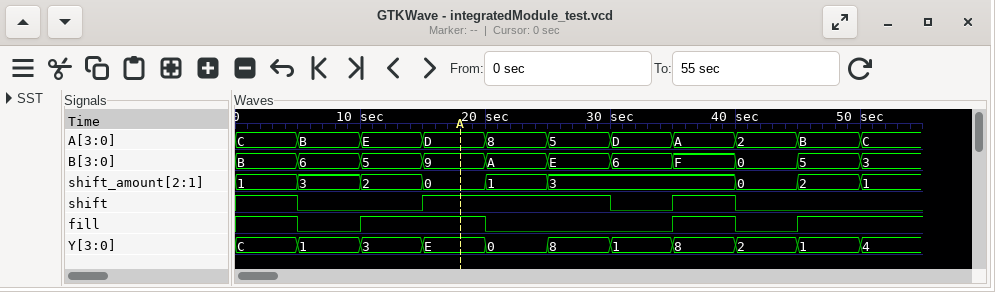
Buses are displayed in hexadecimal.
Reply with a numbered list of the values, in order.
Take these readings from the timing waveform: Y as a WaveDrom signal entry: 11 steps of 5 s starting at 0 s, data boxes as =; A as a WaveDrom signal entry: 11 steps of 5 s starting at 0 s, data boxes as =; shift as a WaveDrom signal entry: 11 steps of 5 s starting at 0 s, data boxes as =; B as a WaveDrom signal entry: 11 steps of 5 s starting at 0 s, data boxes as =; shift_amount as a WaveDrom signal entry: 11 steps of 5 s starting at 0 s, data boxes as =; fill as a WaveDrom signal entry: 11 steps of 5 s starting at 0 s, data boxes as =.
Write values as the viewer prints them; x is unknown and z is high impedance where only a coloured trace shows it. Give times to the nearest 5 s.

1. {name: 'Y', wave: '===========', data: 'C 1 3 E 0 8 1 8 2 1 4'}
2. {name: 'A', wave: '===========', data: 'C B E D 8 5 D A 2 B C'}
3. {name: 'shift', wave: '10.1..010..'}
4. {name: 'B', wave: '===========', data: 'B 6 5 9 A E 6 F 0 5 3'}
5. {name: 'shift_amount', wave: '======..===', data: '1 3 2 0 1 3 0 2 1'}
6. {name: 'fill', wave: '101.0..101.'}
